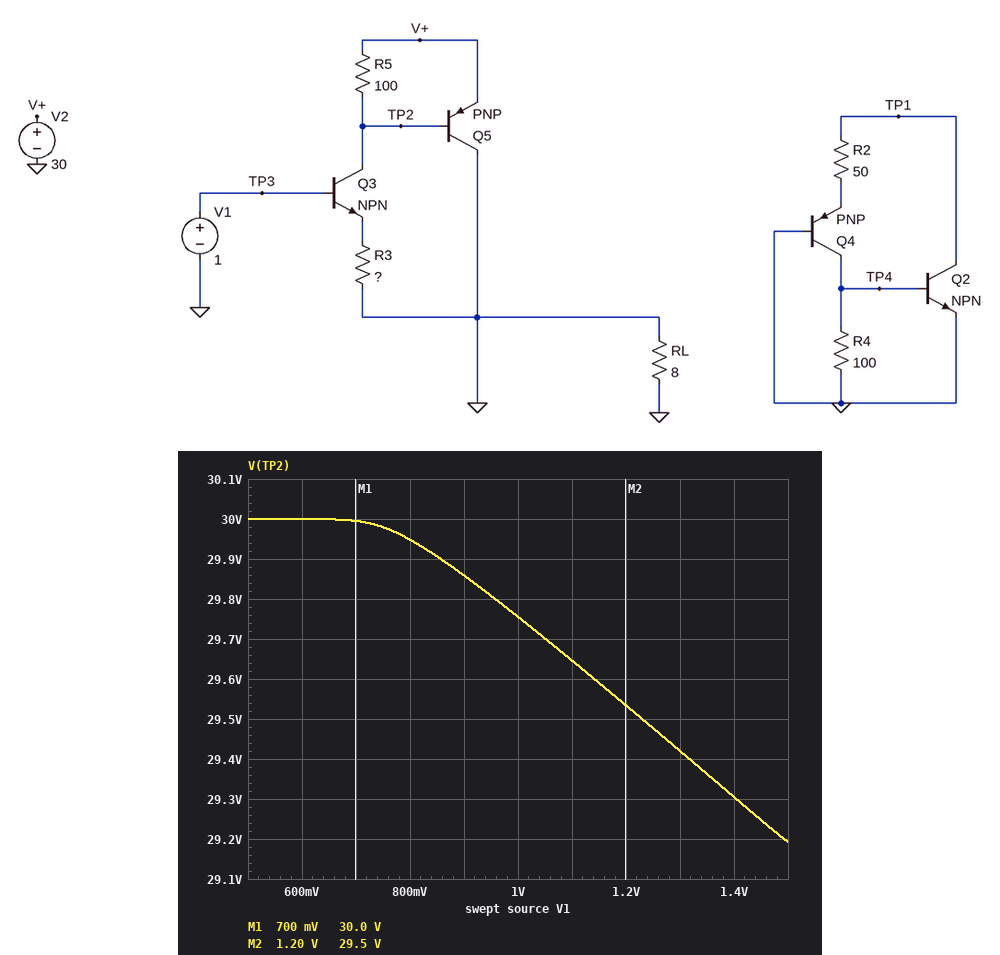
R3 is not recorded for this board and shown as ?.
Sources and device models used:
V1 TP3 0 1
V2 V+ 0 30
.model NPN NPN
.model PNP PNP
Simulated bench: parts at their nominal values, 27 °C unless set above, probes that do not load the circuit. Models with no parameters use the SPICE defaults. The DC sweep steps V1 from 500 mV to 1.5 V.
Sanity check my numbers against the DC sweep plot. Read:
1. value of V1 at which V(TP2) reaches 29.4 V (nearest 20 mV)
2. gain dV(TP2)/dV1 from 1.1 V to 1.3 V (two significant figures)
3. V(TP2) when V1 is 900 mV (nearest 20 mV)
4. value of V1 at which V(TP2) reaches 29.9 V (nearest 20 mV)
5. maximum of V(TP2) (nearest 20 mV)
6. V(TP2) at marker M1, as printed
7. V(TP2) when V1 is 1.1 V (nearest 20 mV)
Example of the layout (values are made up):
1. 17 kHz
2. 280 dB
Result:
1. 1.32 V
2. -1.1 V/V
3. 29.86 V
4. 860 mV
5. 30.00 V
6. 30.0 V
7. 29.64 V
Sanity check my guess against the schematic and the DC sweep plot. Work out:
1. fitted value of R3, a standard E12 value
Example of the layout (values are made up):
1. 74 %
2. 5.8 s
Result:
1. 82 Ω
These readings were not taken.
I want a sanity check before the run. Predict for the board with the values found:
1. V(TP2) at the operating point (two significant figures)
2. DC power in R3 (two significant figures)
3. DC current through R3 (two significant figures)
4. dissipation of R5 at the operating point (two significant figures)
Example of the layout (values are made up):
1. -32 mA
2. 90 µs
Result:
1. 30 V
2. 500 µW
3. 2.5 mA
4. 600 µW
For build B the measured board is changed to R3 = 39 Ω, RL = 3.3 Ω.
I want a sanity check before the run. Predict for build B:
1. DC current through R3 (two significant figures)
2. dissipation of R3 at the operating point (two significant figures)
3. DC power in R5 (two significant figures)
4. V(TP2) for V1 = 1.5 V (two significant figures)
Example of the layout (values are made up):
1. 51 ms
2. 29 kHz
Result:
1. 4.8 mA
2. 880 µW
3. 2.2 mW
4. 29 V
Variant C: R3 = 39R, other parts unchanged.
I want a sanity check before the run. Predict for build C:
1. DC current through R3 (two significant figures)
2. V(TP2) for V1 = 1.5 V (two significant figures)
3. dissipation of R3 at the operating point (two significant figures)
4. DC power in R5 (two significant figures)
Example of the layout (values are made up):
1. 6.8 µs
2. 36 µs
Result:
1. 4.8 mA
2. 29 V
3. 880 µW
4. 2.2 mW
